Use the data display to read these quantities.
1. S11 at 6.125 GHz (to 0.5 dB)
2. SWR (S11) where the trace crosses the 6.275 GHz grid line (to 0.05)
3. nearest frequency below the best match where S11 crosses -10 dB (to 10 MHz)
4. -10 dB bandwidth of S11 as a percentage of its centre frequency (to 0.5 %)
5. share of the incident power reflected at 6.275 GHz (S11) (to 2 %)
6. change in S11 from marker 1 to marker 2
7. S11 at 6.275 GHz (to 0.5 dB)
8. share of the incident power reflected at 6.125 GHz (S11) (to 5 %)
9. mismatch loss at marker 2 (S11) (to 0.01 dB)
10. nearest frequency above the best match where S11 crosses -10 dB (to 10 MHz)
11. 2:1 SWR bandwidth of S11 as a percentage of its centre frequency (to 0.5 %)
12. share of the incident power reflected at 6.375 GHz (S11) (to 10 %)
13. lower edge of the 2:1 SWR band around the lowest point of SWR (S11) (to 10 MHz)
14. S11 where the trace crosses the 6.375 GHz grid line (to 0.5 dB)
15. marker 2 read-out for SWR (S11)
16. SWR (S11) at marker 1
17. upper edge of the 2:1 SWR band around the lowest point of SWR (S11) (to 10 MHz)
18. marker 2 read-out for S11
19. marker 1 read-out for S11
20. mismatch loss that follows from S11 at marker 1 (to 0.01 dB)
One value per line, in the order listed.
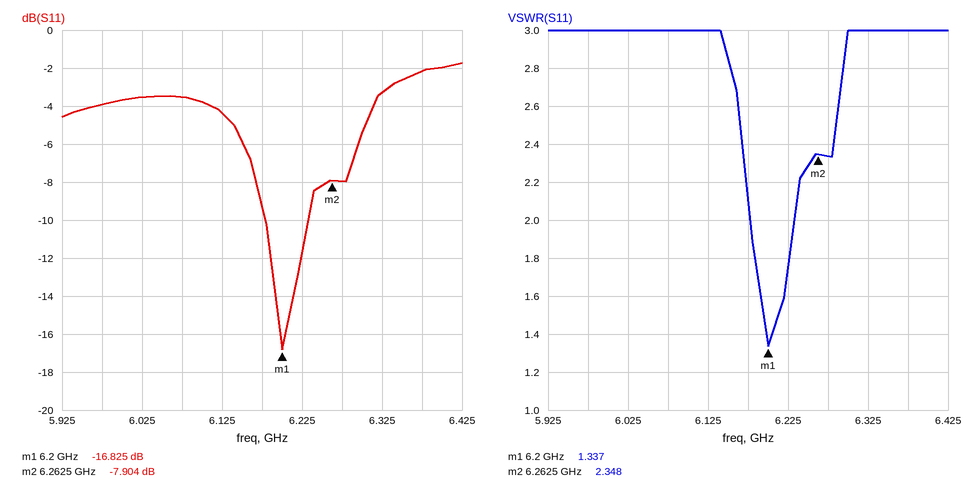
-4.5 dB
2.35
6.18 GHz
1.0 %
16 %
8.921 dB
-8.0 dB
35 %
0.77 dB
6.23 GHz
1.0 %
60 %
6.18 GHz
-2.0 dB
2.348
1.337
6.23 GHz
-7.904 dB
-16.825 dB
0.09 dB
